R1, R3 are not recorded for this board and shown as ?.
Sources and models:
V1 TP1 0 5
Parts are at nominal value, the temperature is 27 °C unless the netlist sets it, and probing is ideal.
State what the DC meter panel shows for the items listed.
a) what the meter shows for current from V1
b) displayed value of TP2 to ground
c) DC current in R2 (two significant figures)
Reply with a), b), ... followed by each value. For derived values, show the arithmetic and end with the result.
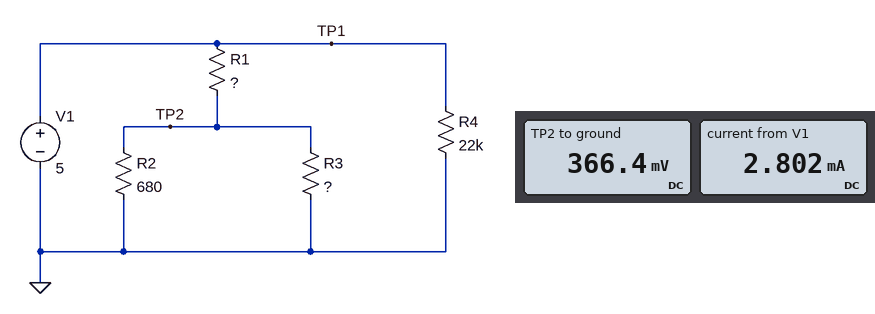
a) 2.802 mA
b) 366.4 mV
c) (366.4 mV) / 680 Ω = 540 µA
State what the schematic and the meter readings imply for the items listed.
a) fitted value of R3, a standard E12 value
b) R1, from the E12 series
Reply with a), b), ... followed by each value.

a) 180 Ω
b) 1.8 kΩ
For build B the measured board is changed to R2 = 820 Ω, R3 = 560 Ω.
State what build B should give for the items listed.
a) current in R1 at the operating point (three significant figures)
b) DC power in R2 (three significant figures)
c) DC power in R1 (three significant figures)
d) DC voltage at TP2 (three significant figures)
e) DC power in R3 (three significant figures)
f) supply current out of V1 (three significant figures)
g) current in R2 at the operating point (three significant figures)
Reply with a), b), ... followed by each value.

a) 2.34 mA
b) 742 µW
c) 9.89 mW
d) 780 mV
e) 1.09 mW
f) 2.57 mA
g) 951 µA
